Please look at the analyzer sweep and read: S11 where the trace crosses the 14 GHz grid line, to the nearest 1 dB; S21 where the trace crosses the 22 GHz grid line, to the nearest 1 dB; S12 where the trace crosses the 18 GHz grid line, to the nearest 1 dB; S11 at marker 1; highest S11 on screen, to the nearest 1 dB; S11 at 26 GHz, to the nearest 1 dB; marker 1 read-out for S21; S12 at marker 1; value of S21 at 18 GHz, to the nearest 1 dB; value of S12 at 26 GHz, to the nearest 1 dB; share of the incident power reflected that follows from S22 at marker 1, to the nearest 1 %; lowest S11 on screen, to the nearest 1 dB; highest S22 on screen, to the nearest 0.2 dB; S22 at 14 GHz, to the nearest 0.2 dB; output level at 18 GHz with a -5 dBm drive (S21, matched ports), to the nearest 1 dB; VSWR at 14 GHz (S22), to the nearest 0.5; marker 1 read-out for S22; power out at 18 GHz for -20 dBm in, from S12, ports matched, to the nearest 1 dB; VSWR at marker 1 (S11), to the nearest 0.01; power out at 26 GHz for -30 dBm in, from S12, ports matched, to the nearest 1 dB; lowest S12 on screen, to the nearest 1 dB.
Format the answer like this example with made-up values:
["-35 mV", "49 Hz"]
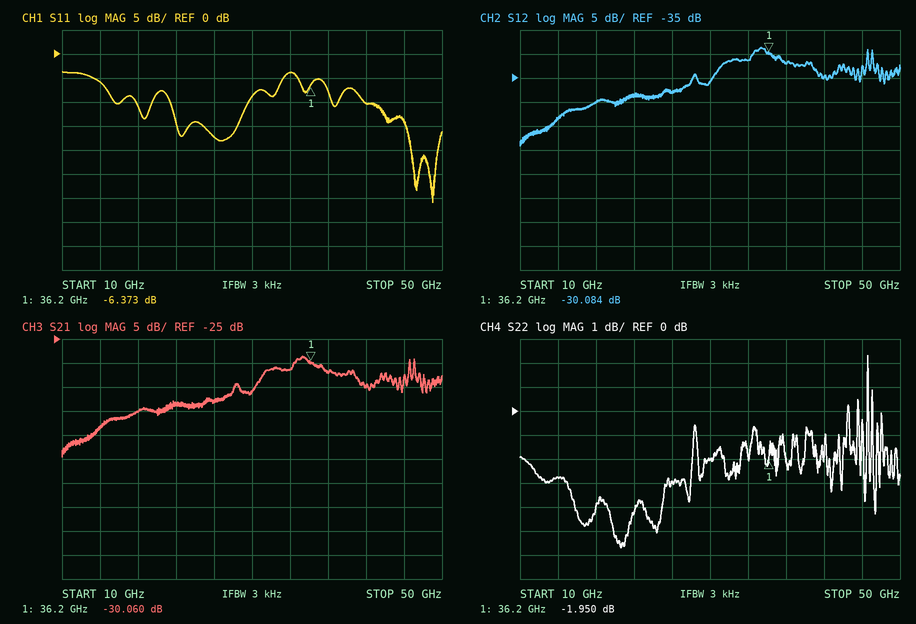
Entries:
["-6 dB", "-38 dB", "-40 dB", "-6.373 dB", "-4 dB", "-17 dB", "-30.060 dB", "-30.084 dB", "-40 dB", "-38 dB", "64 %", "-31 dB", "2.4 dB", "-2.8 dB", "-45 dBm", "6.5", "-1.950 dB", "-60 dBm", "2.85", "-68 dBm", "-49 dB"]
